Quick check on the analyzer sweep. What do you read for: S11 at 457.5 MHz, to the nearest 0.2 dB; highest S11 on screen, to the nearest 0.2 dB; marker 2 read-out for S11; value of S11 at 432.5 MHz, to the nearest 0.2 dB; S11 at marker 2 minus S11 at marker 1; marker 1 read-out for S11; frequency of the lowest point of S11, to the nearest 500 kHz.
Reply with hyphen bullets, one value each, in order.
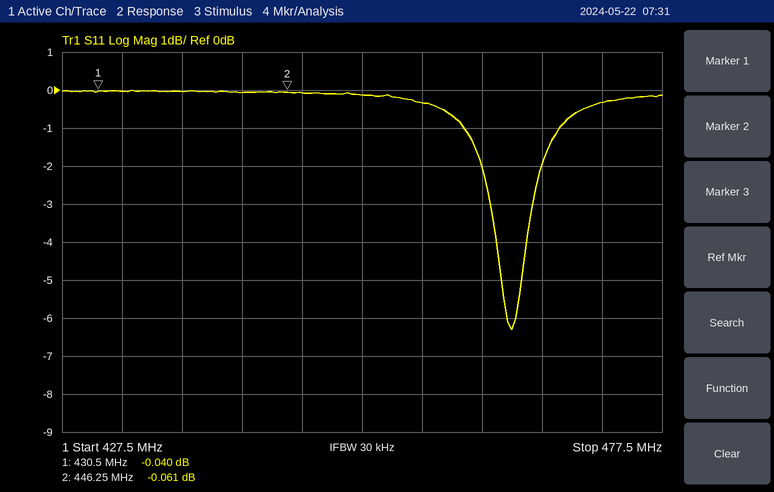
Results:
- -0.4 dB
- 0.0 dB
- -0.061 dB
- 0.0 dB
- -0.021 dB
- -0.040 dB
- 465.0 MHz
